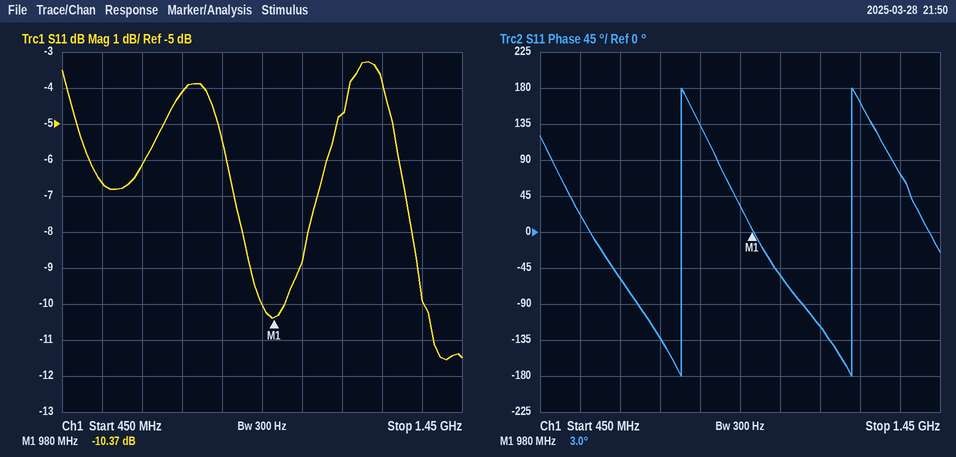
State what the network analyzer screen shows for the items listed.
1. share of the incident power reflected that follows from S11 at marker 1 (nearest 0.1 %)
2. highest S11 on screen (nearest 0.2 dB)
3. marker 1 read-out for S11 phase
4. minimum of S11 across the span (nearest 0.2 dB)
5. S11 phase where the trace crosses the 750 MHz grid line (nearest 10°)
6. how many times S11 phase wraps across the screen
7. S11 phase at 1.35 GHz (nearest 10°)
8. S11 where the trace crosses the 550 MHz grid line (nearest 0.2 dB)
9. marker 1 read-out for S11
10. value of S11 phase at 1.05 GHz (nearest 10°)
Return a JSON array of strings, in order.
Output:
["9.2 %", "-3.2 dB", "3.0°", "-11.6 dB", "-130°", "2", "70°", "-6.6 dB", "-10.37 dB", "-50°"]
